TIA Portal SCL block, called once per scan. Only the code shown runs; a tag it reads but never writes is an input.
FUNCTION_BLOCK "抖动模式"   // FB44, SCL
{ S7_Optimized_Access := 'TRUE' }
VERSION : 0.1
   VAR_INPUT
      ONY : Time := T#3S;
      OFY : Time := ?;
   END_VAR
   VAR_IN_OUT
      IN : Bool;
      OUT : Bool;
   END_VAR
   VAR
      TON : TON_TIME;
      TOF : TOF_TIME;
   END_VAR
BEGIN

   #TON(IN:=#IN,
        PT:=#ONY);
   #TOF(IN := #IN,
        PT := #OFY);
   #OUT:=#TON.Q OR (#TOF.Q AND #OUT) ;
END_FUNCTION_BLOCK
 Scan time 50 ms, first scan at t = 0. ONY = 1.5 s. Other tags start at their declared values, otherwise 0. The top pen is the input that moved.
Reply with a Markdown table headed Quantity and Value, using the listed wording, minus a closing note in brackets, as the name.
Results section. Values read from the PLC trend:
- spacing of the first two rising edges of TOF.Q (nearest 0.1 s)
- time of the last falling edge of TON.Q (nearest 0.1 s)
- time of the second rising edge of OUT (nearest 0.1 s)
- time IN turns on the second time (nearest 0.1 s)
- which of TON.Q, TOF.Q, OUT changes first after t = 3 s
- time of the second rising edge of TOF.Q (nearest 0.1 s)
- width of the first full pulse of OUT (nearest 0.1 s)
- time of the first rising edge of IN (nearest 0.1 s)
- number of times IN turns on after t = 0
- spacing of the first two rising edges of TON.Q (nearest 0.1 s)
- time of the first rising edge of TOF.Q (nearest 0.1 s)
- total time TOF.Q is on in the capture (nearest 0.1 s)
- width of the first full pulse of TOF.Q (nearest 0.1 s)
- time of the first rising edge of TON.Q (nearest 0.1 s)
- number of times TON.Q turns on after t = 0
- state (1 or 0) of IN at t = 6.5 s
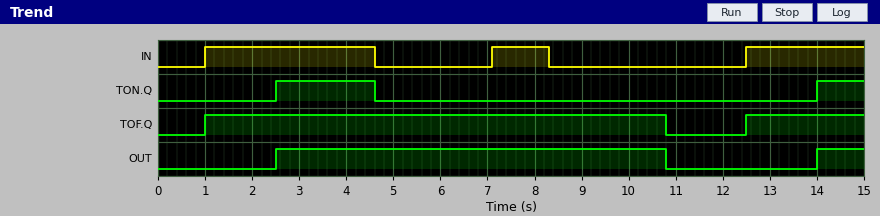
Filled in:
| Quantity | Value |
|---|---|
| spacing of the first two rising edges of TOF.Q | 11.5 s |
| time of the last falling edge of TON.Q | 4.6 s |
| time of the second rising edge of OUT | 14.0 s |
| time IN turns on the second time | 7.1 s |
| which of TON.Q, TOF.Q, OUT changes first after t = 3 s | TON.Q |
| time of the second rising edge of TOF.Q | 12.5 s |
| width of the first full pulse of OUT | 8.3 s |
| time of the first rising edge of IN | 1.0 s |
| number of times IN turns on after t = 0 | 3 |
| spacing of the first two rising edges of TON.Q | 11.5 s |
| time of the first rising edge of TOF.Q | 1.0 s |
| total time TOF.Q is on in the capture | 12.3 s |
| width of the first full pulse of TOF.Q | 9.8 s |
| time of the first rising edge of TON.Q | 2.5 s |
| number of times TON.Q turns on after t = 0 | 2 |
| state (1 or 0) of IN at t = 6.5 s | 0 |
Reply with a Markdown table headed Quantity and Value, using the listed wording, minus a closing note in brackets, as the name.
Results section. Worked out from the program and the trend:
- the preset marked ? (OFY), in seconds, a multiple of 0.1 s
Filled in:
| Quantity | Value |
|---|---|
| the preset marked ? (OFY), in seconds, a multiple of 0.1 s | 2.5 s |
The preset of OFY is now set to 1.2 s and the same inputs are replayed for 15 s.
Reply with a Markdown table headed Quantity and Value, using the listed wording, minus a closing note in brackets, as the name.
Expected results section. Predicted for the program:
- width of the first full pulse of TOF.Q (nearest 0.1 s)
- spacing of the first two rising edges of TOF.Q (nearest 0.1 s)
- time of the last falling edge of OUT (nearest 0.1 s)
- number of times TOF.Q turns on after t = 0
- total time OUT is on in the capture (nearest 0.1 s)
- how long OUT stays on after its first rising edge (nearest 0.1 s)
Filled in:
| Quantity | Value |
|---|---|
| width of the first full pulse of TOF.Q | 4.8 s |
| spacing of the first two rising edges of TOF.Q | 6.1 s |
| time of the last falling edge of OUT | 5.8 s |
| number of times TOF.Q turns on after t = 0 | 3 |
| total time OUT is on in the capture | 4.3 s |
| how long OUT stays on after its first rising edge | 3.3 s |
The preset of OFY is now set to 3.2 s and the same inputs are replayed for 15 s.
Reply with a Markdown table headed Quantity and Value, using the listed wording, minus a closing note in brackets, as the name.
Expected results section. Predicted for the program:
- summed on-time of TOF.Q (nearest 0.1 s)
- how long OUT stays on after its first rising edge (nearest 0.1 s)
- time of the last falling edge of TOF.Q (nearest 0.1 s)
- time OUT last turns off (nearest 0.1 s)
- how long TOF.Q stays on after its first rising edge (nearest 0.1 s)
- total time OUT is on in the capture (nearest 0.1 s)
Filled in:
| Quantity | Value |
|---|---|
| summed on-time of TOF.Q | 13.0 s |
| how long OUT stays on after its first rising edge | 9.0 s |
| time of the last falling edge of TOF.Q | 11.5 s |
| time OUT last turns off | 11.5 s |
| how long TOF.Q stays on after its first rising edge | 10.5 s |
| total time OUT is on in the capture | 10.0 s |
